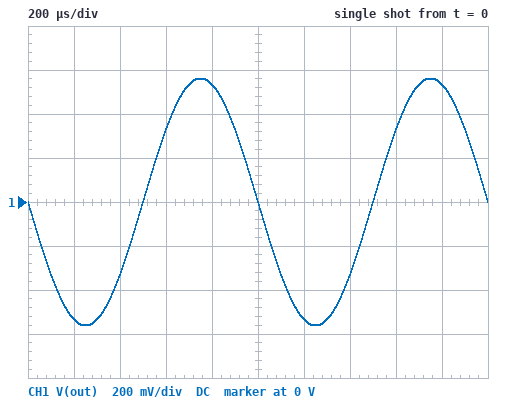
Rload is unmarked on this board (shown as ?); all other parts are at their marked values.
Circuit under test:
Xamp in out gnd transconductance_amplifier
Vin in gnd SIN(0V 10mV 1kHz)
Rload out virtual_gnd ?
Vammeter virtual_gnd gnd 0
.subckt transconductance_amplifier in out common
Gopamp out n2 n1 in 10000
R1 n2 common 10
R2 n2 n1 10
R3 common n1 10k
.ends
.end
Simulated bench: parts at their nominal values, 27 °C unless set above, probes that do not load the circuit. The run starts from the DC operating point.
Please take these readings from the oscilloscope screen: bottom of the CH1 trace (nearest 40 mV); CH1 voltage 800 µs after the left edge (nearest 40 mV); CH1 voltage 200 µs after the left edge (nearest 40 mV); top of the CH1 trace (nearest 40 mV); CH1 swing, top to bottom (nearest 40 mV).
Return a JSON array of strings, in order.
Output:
["-560 mV", "520 mV", "-520 mV", "560 mV", "1.12 V"]
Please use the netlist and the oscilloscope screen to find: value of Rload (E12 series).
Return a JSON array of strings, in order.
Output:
["560 Ω"]
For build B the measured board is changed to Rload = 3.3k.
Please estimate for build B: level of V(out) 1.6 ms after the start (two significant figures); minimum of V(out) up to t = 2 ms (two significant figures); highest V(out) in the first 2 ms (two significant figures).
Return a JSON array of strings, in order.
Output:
["1.9 V", "-3.3 V", "3.3 V"]
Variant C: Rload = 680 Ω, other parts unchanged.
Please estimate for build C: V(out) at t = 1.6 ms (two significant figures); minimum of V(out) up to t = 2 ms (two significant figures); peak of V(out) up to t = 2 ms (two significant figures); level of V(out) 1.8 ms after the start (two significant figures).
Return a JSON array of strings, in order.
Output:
["400 mV", "-680 mV", "680 mV", "650 mV"]
